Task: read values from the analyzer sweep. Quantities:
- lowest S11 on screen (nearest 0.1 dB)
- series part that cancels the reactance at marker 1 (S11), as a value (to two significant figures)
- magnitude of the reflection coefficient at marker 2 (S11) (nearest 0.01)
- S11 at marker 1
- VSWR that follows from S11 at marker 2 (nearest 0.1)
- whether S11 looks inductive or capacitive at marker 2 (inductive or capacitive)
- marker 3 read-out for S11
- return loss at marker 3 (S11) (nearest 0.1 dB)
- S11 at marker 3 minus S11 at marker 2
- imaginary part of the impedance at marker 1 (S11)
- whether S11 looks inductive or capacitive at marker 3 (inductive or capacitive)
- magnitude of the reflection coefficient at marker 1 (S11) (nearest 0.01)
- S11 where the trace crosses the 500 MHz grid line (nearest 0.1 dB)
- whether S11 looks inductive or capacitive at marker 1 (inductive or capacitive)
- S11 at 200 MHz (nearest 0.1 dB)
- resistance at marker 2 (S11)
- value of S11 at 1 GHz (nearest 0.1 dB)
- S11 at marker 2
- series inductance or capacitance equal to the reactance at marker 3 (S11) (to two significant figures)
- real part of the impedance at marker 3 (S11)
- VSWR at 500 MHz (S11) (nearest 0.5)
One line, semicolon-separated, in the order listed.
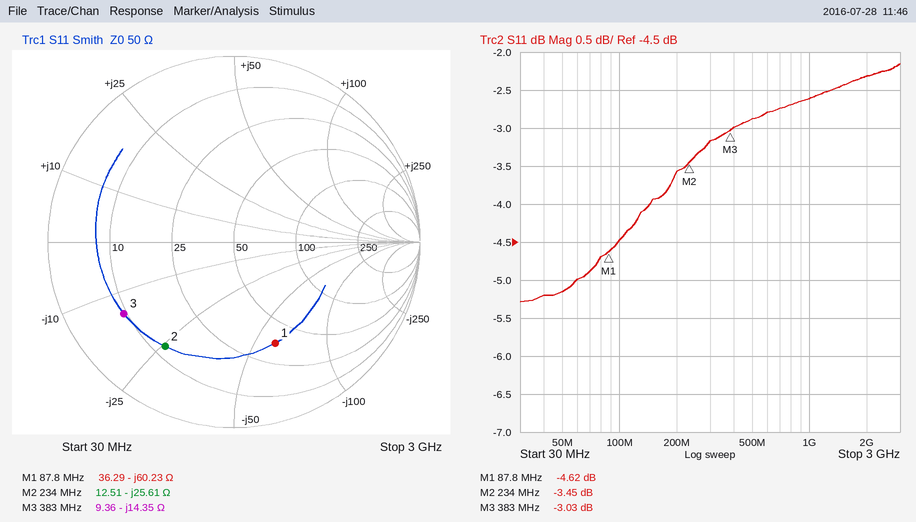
-5.3 dB; 110 nH; 0.67; -4.62 dB; 5.1; capacitive; -3.03 dB; 3.0 dB; 0.42 dB; -60.23 Ω; capacitive; 0.59; -2.9 dB; capacitive; -3.6 dB; 12.51 Ω; -2.6 dB; -3.45 dB; 29 pF; 9.36 Ω; 6.0
